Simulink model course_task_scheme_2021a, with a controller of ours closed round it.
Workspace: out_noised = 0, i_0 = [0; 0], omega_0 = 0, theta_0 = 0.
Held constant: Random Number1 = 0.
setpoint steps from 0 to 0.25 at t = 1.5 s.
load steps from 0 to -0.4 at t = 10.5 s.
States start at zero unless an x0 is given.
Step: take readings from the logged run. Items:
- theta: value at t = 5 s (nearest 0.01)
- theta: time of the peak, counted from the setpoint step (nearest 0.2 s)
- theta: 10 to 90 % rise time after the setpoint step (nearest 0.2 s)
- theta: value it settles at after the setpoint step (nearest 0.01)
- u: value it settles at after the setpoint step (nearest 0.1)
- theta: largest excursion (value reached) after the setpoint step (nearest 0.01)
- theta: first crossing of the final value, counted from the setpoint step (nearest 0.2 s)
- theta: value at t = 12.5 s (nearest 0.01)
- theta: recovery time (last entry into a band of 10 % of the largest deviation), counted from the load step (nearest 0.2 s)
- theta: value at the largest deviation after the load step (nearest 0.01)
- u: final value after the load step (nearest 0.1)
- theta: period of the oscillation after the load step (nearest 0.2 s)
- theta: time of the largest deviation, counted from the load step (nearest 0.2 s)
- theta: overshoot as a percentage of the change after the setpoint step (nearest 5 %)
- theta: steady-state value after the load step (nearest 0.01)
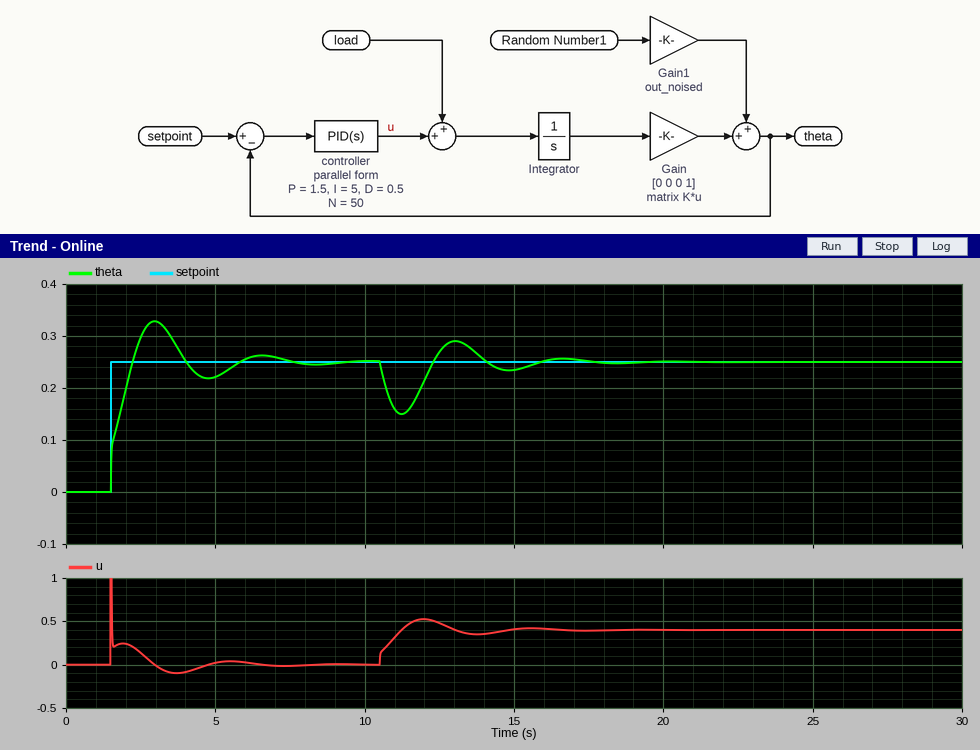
0.22
1.4 s
0.6 s
0.25
0.0
0.33
0.8 s
0.27
4.8 s
0.15
0.4
3.6 s
0.8 s
30 %
0.25
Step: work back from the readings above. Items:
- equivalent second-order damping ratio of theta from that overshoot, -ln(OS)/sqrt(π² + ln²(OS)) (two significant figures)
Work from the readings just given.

0.36
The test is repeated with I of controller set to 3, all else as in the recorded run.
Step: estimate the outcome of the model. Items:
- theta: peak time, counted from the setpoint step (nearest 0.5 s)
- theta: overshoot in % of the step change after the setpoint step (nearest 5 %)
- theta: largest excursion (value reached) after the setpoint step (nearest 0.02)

2.0 s
25 %
0.32
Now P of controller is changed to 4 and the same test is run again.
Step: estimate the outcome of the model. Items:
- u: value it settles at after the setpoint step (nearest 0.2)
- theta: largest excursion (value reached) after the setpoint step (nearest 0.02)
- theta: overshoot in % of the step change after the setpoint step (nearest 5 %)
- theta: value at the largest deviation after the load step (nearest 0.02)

0.0
0.28
15 %
0.18
